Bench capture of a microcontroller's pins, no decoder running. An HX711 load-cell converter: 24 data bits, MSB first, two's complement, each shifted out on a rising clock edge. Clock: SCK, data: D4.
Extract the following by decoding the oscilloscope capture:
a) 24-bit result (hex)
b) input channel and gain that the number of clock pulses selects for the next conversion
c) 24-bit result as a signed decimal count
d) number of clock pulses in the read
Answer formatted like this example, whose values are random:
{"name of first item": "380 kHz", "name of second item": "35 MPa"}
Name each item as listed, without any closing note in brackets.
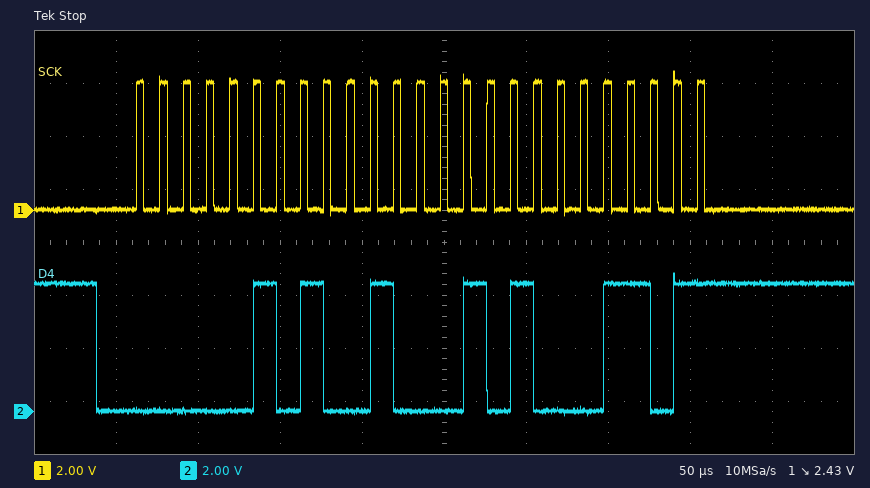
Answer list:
{"24-bit result": "0x05228D", "input channel and gain that the number of clock pulses selects for the next conversion": "channel A, gain 128", "24-bit result as a signed decimal count": "336525", "number of clock pulses in the read": "25"}
